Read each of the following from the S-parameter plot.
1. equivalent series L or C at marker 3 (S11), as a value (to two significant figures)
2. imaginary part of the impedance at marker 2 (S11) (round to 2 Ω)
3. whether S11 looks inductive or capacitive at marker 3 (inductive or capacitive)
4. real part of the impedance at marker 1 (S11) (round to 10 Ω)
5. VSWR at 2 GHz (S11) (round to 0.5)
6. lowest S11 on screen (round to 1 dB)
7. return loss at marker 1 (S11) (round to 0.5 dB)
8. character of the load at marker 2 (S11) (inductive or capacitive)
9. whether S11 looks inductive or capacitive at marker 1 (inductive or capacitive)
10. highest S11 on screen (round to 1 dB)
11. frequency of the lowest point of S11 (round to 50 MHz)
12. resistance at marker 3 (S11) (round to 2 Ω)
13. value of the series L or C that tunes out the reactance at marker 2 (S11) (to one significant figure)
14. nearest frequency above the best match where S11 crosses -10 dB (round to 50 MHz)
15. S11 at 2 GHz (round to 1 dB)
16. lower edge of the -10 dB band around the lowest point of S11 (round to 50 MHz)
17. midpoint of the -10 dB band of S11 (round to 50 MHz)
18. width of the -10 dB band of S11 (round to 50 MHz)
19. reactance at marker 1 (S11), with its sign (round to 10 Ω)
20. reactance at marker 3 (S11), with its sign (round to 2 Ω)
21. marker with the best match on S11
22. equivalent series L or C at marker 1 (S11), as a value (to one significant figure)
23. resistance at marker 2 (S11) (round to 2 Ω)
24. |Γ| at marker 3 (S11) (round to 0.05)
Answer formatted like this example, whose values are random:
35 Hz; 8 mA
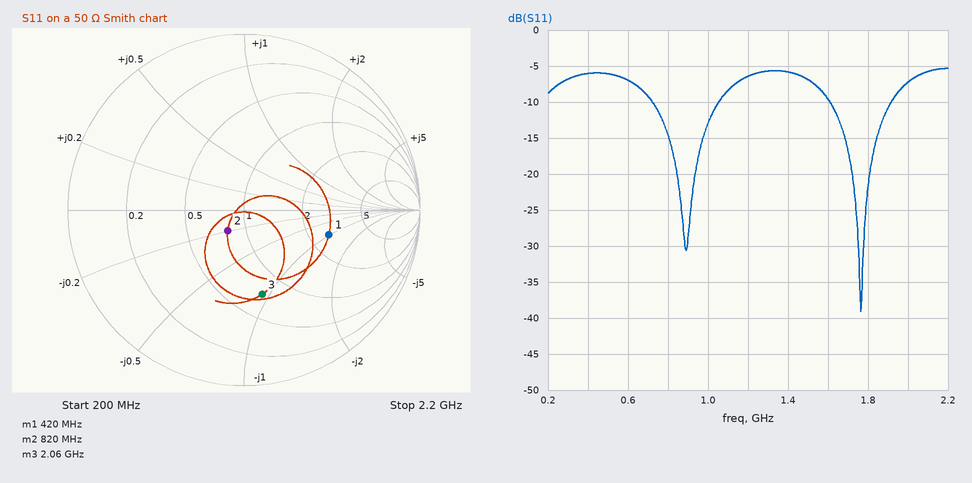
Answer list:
1.7 pF; -10 Ω; capacitive; 130 Ω; 2.5; -39 dB; 6.0 dB; capacitive; capacitive; -5 dB; 1.75 GHz; 36 Ω; 2 nH; 1.90 GHz; -7 dB; 1.60 GHz; 1.75 GHz; 300 MHz; -50 Ω; -46 Ω; marker 2; 8 pF; 40 Ω; 0.50
